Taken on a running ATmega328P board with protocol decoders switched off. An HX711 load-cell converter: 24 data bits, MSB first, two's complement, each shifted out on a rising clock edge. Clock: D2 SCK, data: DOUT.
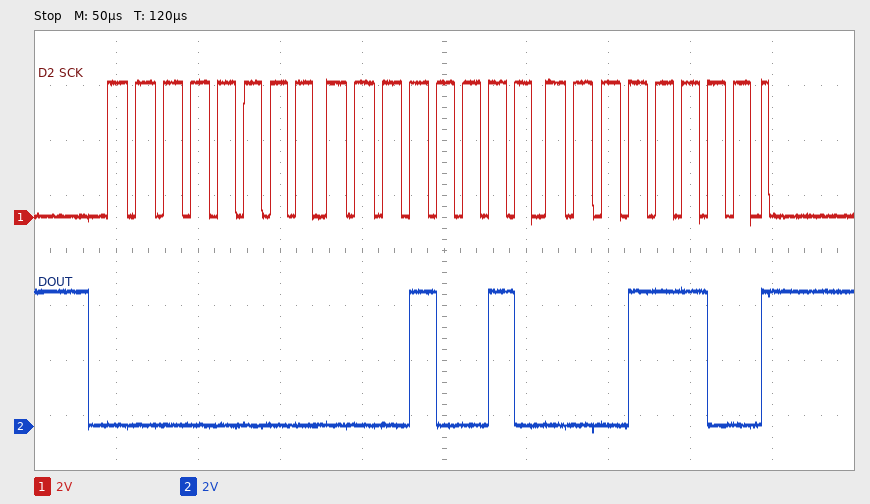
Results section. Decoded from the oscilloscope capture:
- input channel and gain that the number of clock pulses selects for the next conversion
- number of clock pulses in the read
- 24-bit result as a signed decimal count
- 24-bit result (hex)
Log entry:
channel A, gain 128
25
4636
0x00121C
